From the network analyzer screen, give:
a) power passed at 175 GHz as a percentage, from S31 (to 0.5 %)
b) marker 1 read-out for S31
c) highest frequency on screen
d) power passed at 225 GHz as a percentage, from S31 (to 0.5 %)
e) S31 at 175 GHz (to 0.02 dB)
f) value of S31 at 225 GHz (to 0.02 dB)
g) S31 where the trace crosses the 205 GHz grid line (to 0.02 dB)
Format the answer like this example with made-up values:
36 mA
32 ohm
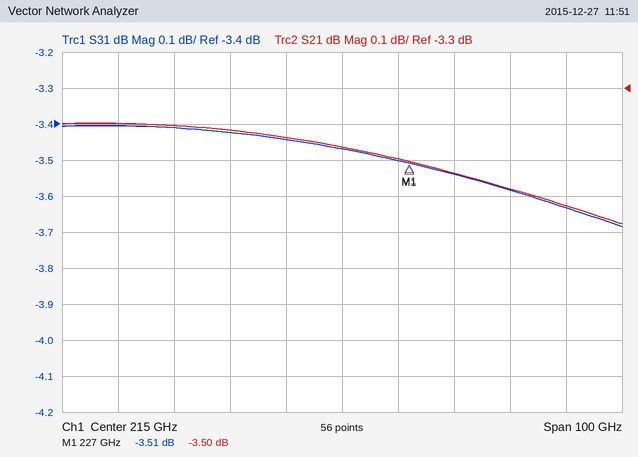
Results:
45.5 %
-3.51 dB
265 GHz
44.5 %
-3.40 dB
-3.50 dB
-3.44 dB
